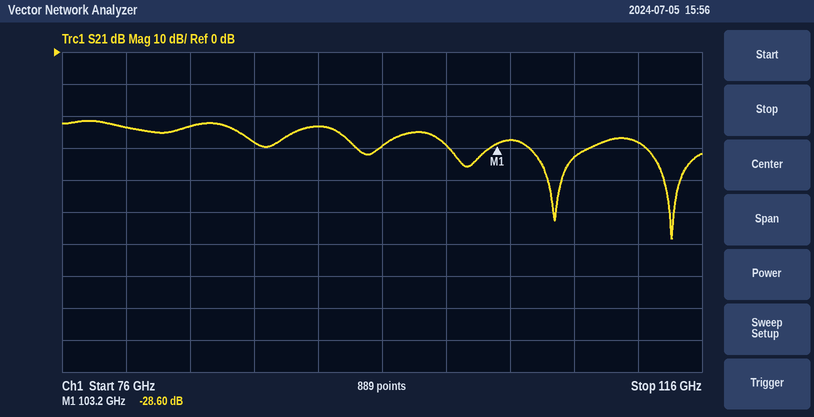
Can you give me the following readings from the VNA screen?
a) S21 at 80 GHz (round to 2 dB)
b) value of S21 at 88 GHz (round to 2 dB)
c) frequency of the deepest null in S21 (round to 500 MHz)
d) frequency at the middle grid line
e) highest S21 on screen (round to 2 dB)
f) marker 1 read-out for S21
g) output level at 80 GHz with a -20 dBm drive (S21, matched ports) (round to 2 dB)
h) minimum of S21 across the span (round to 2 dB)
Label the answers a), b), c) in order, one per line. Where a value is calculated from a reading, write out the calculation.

a) -24 dB
b) -28 dB
c) 114.0 GHz
d) 96 GHz
e) -22 dB
f) -28.60 dB
g) -20 dBm + (-24 dB) = -44 dBm
h) -58 dB
